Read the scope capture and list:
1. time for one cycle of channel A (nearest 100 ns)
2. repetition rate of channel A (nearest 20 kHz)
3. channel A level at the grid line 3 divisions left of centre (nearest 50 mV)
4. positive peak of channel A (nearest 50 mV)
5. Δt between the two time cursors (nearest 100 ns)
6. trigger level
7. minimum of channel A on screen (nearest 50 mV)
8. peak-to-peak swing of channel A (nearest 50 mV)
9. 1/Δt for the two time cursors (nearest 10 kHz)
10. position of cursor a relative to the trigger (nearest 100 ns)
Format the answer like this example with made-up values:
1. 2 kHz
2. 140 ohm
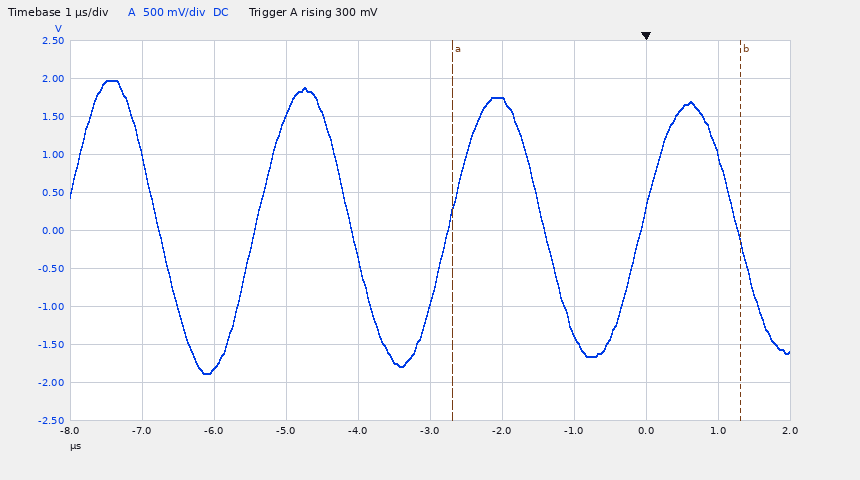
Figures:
1. 2.7 µs
2. 380 kHz
3. -1.80 V
4. 1.95 V
5. 4.0 µs
6. 300 mV
7. -1.90 V
8. 3.85 V
9. 250 kHz
10. -2.7 µs
